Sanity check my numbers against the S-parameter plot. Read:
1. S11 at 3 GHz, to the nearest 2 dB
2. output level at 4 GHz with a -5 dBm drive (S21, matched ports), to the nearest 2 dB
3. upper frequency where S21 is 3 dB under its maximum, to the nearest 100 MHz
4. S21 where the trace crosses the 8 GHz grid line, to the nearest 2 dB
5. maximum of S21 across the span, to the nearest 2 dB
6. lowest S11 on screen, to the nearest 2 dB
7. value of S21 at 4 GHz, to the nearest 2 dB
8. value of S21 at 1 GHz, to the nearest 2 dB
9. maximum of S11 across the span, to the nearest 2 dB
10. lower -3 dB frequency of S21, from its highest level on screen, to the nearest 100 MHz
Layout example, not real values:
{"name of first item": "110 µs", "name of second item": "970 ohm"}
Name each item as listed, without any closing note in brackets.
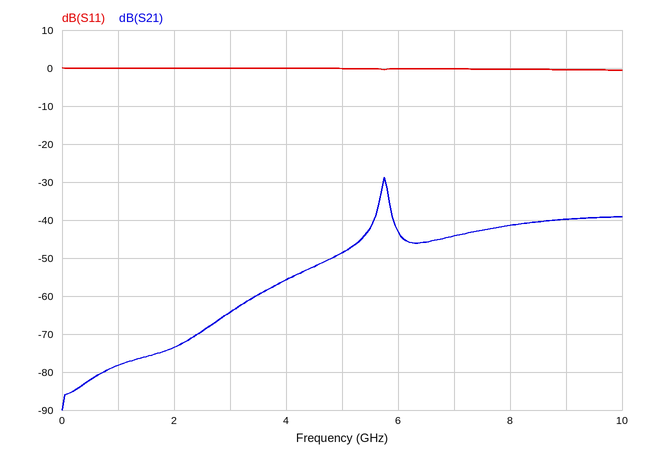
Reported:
{"S11 at 3 GHz, to the nearest 2 dB": "0 dB", "output level at 4 GHz with a -5 dBm drive (S21, matched ports), to the nearest 2 dB": "-60 dBm", "upper frequency where S21 is 3 dB under its maximum, to the nearest 100 MHz": "5.8 GHz", "S21 where the trace crosses the 8 GHz grid line, to the nearest 2 dB": "-42 dB", "maximum of S21 across the span, to the nearest 2 dB": "-28 dB", "lowest S11 on screen, to the nearest 2 dB": "0 dB", "value of S21 at 4 GHz, to the nearest 2 dB": "-56 dB", "value of S21 at 1 GHz, to the nearest 2 dB": "-78 dB", "maximum of S11 across the span, to the nearest 2 dB": "0 dB", "lower -3 dB frequency of S21, from its highest level on screen, to the nearest 100 MHz": "5.7 GHz"}
